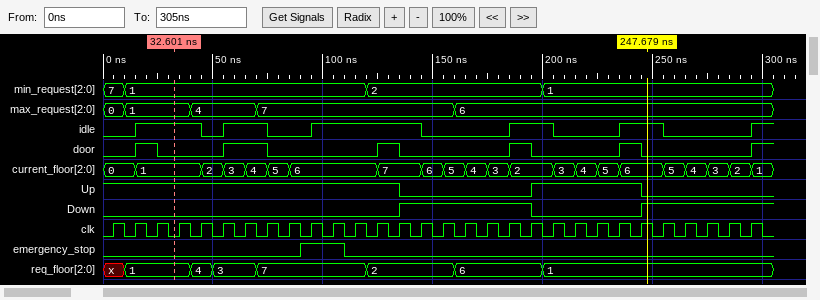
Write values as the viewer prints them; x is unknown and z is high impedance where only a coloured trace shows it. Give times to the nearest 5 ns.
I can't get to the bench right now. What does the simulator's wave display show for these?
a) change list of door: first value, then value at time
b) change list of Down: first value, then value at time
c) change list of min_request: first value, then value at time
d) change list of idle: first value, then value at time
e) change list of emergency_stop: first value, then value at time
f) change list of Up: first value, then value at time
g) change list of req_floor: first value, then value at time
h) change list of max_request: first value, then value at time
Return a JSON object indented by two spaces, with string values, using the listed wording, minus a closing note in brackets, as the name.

{
  "change list of door: first value, then value at time": "0, 1 at 15 ns, 0 at 25 ns, 1 at 55 ns, 0 at 75 ns, 1 at 125 ns, 0 at 135 ns, 1 at 185 ns, 0 at 195 ns, 1 at 235 ns, 0 at 245 ns, 1 at 295 ns",
  "change list of Down: first value, then value at time": "0, 1 at 135 ns, 0 at 195 ns, 1 at 245 ns",
  "change list of min_request: first value, then value at time": "7, 1 at 10 ns, 2 at 120 ns, 1 at 200 ns",
  "change list of idle: first value, then value at time": "0, 1 at 15 ns, 0 at 45 ns, 1 at 55 ns, 0 at 75 ns, 1 at 95 ns, 0 at 145 ns, 1 at 185 ns, 0 at 205 ns, 1 at 235 ns, 0 at 255 ns, 1 at 295 ns",
  "change list of emergency_stop: first value, then value at time": "0, 1 at 90 ns, 0 at 110 ns",
  "change list of Up: first value, then value at time": "1, 0 at 135 ns, 1 at 195 ns, 0 at 245 ns",
  "change list of req_floor: first value, then value at time": "x, 1 at 10 ns, 4 at 40 ns, 3 at 50 ns, 7 at 70 ns, 2 at 120 ns, 6 at 160 ns, 1 at 200 ns",
  "change list of max_request: first value, then value at time": "0, 1 at 10 ns, 4 at 40 ns, 7 at 70 ns, 6 at 160 ns"
}
